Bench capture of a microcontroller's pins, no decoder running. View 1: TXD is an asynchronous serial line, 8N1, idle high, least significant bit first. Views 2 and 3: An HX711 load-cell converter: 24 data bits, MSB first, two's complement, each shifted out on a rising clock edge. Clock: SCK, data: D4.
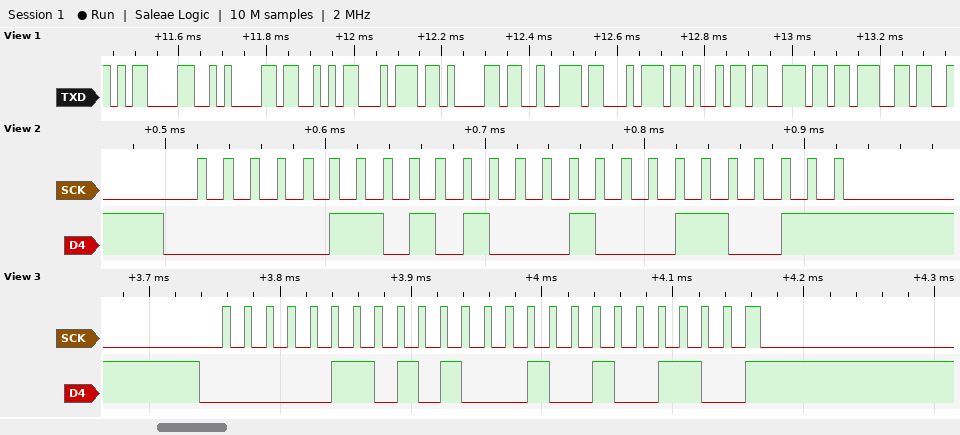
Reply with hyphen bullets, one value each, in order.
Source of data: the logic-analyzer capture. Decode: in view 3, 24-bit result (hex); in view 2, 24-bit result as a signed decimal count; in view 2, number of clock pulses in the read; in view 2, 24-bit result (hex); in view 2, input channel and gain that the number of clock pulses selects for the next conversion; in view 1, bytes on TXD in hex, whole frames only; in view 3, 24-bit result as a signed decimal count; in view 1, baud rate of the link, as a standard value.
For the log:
- 0x06A24C
- 434739
- 25
- 0x06A233
- channel A, gain 128
- 0D 0A 53 74 61 72 74 69 6E 67
- 434764
- 57600 baud
